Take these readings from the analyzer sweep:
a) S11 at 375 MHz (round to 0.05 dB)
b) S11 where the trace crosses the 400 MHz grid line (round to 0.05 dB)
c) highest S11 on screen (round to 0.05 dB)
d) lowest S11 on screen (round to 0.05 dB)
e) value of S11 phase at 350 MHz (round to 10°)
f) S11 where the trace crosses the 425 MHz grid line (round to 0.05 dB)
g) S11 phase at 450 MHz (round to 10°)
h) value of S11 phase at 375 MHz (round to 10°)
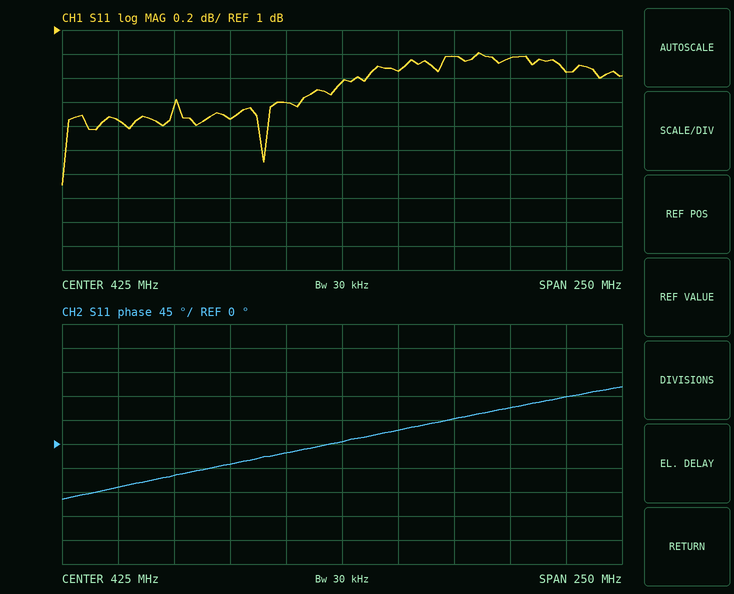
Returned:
0.25 dB
0.40 dB
0.80 dB
-0.30 dB
-60°
0.55 dB
30°
-40°
